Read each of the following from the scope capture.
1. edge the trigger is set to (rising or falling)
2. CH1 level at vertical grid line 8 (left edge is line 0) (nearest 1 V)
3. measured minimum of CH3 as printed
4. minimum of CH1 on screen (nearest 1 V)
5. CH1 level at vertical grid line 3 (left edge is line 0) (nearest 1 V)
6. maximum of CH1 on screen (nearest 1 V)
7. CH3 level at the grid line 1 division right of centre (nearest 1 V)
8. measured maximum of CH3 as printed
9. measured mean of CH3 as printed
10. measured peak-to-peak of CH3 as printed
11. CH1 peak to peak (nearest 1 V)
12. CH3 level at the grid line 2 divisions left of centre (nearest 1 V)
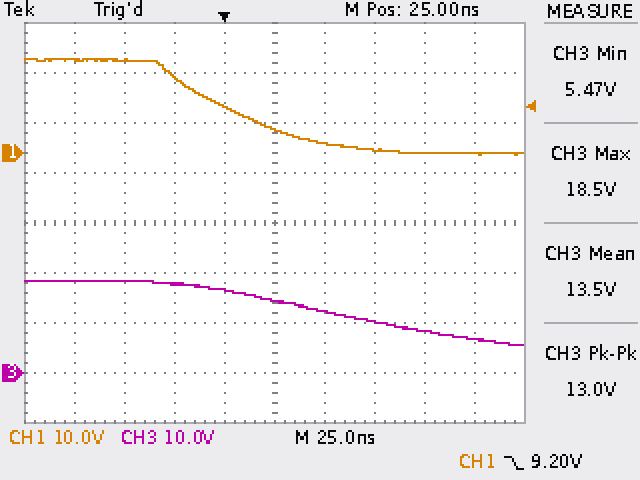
falling
0 V
5.47 V
0 V
15 V
19 V
12 V
18.5 V
13.5 V
13.0 V
19 V
18 V
